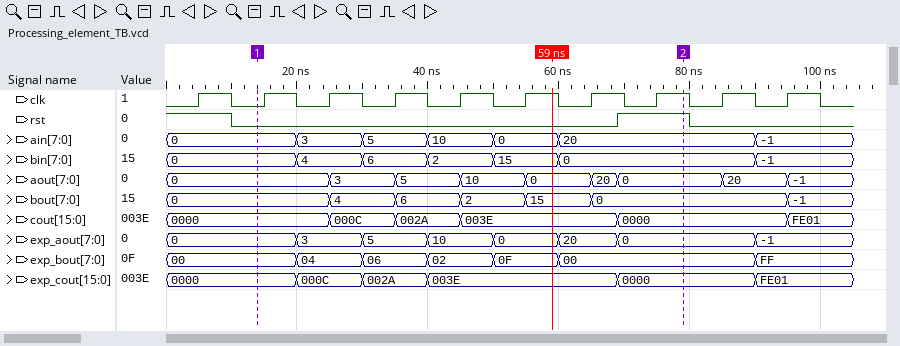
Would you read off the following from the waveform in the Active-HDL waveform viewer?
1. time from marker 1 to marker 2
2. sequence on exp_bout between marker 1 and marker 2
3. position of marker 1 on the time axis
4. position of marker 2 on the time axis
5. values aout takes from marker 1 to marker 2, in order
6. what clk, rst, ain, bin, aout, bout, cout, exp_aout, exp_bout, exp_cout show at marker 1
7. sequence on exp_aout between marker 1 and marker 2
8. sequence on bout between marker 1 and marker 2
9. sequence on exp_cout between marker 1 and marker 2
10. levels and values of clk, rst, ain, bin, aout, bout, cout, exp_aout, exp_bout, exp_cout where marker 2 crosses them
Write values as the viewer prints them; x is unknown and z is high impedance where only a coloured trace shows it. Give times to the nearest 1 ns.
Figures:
65 ns
00, 04, 06, 02, 0F, 00
14 ns
79 ns
0, 3, 5, 10, 0, 20, 0
clk=0, rst=0, ain=0, bin=0, aout=0, bout=0, cout=0000, exp_aout=0, exp_bout=00, exp_cout=0000
0, 3, 5, 10, 0, 20, 0
0, 4, 6, 2, 15, 0
0000, 000C, 002A, 003E, 0000
clk=1, rst=1, ain=20, bin=0, aout=0, bout=0, cout=0000, exp_aout=0, exp_bout=00, exp_cout=0000
